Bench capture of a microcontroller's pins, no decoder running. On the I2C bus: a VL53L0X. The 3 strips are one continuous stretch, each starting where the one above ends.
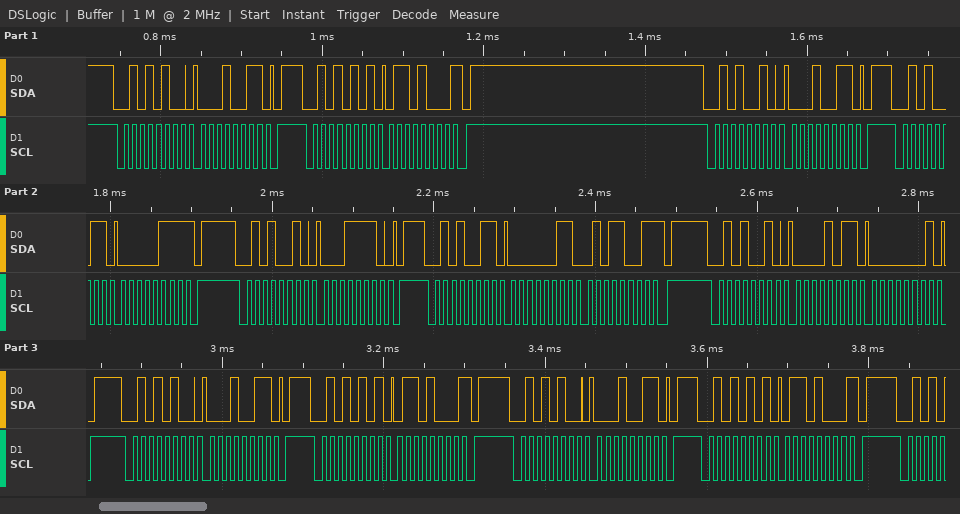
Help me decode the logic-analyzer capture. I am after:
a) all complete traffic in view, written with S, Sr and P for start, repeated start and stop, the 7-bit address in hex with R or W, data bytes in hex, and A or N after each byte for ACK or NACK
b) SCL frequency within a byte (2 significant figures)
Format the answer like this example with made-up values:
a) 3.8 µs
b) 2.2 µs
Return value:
a) S 2AW A 13 A P S 2AR A 68 N P S 29W A 13 A P S 29R A 07 N P S 29W A 1E A P S 29R A 03 A 59 N P S 29W A 0B A 01 A P S 2AW A 13 A P S 2AR A 68 N P S 2AW A 13 A P S 2AR A 68 N P
b) 100 kHz
